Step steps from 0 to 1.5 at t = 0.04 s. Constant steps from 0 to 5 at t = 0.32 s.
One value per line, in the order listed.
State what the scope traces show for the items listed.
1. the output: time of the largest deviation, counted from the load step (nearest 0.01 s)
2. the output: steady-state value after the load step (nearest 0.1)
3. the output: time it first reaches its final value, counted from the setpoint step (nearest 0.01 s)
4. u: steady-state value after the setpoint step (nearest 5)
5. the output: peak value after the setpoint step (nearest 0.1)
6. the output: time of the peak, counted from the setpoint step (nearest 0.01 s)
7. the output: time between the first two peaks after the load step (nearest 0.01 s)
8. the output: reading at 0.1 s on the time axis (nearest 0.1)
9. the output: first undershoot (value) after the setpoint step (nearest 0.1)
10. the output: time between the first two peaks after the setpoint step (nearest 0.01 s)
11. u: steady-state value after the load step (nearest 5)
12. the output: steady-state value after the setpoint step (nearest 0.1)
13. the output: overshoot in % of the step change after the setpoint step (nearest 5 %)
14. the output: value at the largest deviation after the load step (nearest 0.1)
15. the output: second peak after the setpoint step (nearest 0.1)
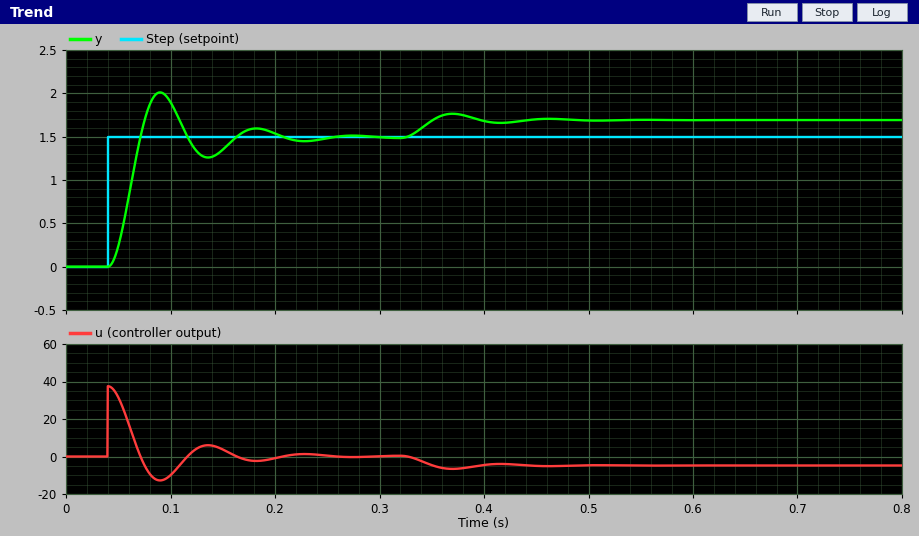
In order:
0.05 s
1.7
0.03 s
0
2.0
0.05 s
0.09 s
1.9
1.3
0.09 s
-5
1.5
35 %
1.8
1.6
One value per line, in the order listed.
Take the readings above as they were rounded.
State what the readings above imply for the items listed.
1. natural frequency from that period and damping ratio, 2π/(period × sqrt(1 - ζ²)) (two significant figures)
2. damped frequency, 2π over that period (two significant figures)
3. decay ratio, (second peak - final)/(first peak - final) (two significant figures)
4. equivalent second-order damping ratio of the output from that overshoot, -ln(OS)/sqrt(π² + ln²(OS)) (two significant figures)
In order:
74 rad/s
70 rad/s
0.20
0.32
